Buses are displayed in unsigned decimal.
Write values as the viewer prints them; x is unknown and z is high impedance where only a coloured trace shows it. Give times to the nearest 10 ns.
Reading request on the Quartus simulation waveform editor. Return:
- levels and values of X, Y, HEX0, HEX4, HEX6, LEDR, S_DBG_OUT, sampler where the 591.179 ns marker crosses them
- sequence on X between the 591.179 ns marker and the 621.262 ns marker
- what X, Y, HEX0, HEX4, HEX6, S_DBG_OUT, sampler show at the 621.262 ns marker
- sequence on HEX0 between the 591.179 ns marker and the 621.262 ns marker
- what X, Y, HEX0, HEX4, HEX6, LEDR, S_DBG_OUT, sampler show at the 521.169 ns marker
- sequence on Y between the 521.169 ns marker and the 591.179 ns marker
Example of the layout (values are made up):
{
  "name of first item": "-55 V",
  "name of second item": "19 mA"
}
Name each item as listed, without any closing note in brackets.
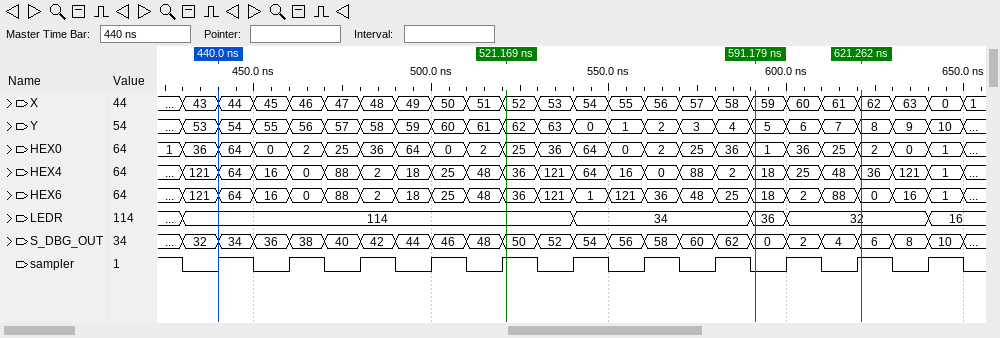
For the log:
{
  "levels and values of X, Y, HEX0, HEX4, HEX6, LEDR, S_DBG_OUT, sampler where the 591.179 ns marker crosses them": "X=59, Y=5, HEX0=1, HEX4=18, HEX6=18, LEDR=36, S_DBG_OUT=0, sampler=0",
  "sequence on X between the 591.179 ns marker and the 621.262 ns marker": "59, 60, 61, 62",
  "what X, Y, HEX0, HEX4, HEX6, S_DBG_OUT, sampler show at the 621.262 ns marker": "X=62, Y=8, HEX0=2, HEX4=36, HEX6=0, S_DBG_OUT=6, sampler=1",
  "sequence on HEX0 between the 591.179 ns marker and the 621.262 ns marker": "1, 36, 25, 2",
  "what X, Y, HEX0, HEX4, HEX6, LEDR, S_DBG_OUT, sampler show at the 521.169 ns marker": "X=52, Y=62, HEX0=25, HEX4=36, HEX6=36, LEDR=114, S_DBG_OUT=50, sampler=1",
  "sequence on Y between the 521.169 ns marker and the 591.179 ns marker": "62, 63, 0, 1, 2, 3, 4, 5"
}
